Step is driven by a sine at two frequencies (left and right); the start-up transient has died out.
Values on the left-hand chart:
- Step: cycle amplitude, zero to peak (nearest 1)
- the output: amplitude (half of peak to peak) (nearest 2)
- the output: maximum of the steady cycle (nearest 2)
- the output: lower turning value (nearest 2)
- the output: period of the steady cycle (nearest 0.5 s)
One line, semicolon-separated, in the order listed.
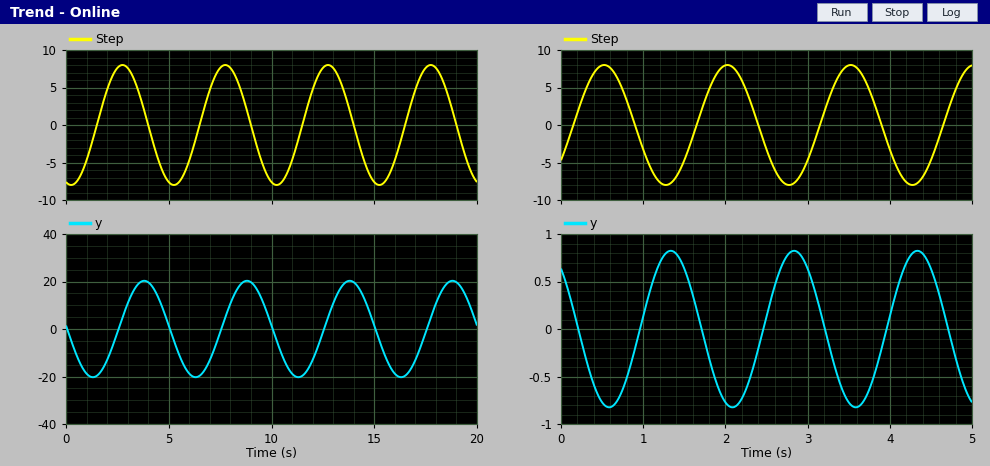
8; 20; 20; -20; 5.0 s
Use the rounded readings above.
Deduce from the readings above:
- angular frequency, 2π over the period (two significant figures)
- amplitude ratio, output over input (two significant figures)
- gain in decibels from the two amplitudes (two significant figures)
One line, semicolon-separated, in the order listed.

1.3 rad/s; 2.5; 8.0 dB
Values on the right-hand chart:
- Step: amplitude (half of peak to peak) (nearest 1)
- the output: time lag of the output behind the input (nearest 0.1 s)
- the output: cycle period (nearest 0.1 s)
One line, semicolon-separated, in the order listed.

8; 0.8 s; 1.5 s
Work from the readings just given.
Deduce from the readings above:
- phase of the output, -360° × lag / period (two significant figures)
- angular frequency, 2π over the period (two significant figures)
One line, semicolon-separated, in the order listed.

-190°; 4.2 rad/s
